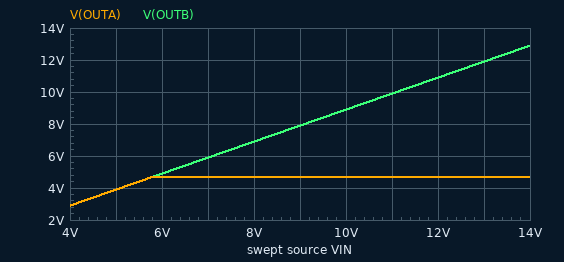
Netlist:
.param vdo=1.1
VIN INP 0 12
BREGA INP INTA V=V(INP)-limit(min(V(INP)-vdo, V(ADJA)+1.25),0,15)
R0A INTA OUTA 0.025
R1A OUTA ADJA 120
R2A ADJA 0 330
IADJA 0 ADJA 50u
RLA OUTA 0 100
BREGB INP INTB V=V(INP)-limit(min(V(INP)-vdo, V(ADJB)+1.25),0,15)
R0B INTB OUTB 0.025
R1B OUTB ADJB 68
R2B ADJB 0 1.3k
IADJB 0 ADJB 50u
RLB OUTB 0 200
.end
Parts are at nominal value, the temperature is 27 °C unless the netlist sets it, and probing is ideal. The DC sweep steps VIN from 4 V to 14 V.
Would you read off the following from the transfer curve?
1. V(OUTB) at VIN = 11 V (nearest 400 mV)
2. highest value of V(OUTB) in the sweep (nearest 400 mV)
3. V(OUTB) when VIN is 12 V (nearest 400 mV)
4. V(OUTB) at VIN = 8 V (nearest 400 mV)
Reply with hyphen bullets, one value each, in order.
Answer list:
- 10.0 V
- 12.8 V
- 10.8 V
- 6.8 V
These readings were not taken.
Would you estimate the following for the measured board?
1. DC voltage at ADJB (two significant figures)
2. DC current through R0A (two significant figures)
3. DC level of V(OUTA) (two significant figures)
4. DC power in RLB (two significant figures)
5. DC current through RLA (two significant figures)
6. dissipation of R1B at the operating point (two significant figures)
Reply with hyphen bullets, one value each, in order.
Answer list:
- 10 V
- 57 mA
- 4.7 V
- 590 mW
- 47 mA
- 4.3 mW
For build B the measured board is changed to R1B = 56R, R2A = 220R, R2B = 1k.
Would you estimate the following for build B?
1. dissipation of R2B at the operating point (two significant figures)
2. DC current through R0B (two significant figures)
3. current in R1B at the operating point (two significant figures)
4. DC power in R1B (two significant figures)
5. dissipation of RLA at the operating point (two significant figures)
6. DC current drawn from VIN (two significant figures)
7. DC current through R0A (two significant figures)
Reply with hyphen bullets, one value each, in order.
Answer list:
- 110 mW
- 65 mA
- 10 mA
- 5.9 mW
- 130 mW
- 110 mA
- 46 mA
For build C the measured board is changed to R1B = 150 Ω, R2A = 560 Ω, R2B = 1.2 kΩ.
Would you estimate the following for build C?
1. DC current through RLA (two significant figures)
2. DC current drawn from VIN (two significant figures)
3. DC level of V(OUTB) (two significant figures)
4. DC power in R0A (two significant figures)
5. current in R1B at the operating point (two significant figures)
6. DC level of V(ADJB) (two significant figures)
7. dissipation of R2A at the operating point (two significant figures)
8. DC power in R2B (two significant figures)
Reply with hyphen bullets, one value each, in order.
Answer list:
- 71 mA
- 140 mA
- 11 V
- 170 µW
- 8.0 mA
- 9.7 V
- 61 mW
- 78 mW
